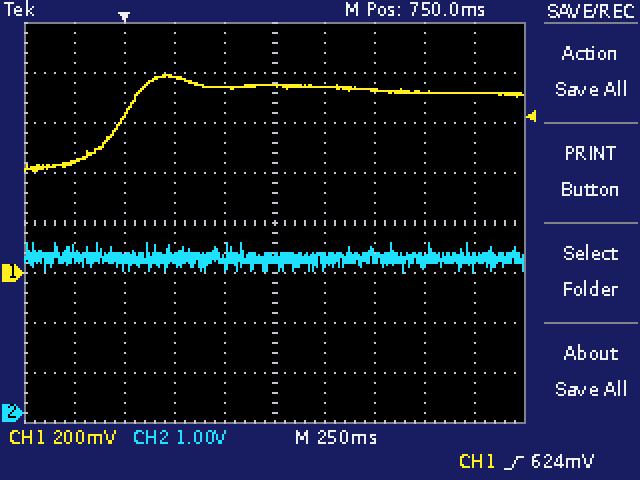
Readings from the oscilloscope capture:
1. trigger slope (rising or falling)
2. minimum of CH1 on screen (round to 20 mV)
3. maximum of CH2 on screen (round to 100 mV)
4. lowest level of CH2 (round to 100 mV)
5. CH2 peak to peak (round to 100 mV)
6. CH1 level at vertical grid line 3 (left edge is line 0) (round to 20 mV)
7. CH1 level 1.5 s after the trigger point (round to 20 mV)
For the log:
rising
400 mV
3.4 V
2.8 V
600 mV
780 mV
720 mV
